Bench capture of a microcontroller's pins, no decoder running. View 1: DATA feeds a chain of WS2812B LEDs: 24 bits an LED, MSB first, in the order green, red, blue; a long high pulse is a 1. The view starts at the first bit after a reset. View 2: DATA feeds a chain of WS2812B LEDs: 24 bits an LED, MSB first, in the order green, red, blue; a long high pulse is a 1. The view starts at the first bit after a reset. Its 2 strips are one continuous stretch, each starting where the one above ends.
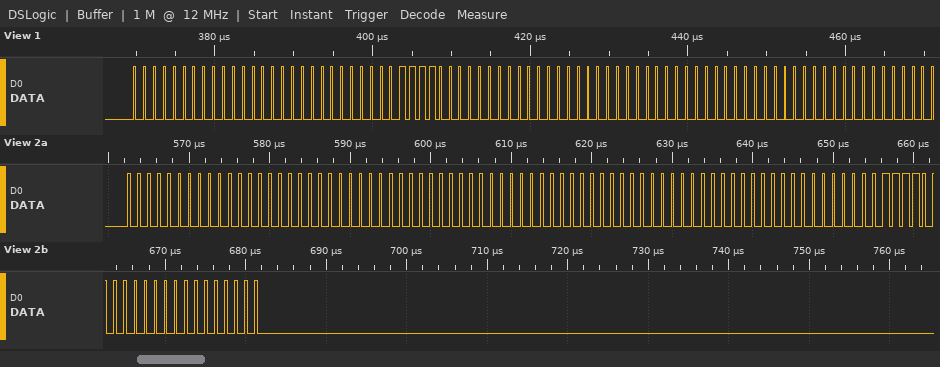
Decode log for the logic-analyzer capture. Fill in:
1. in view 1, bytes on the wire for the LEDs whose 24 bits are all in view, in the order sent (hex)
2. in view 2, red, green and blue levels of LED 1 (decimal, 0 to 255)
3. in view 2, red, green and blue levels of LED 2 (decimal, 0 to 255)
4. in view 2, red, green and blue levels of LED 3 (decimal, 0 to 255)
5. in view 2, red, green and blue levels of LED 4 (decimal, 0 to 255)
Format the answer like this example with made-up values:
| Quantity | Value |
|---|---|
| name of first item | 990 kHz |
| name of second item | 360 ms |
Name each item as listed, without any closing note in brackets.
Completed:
| Quantity | Value |
|---|---|
| in view 1, bytes on the wire for the LEDs whose 24 bits are all in view, in the order sent | 00 00 00 1E 00 00 00 00 00 |
| in view 2, red, green and blue levels of LED 1 | 0, 0, 0 |
| in view 2, red, green and blue levels of LED 2 | 0, 0, 0 |
| in view 2, red, green and blue levels of LED 3 | 0, 0, 0 |
| in view 2, red, green and blue levels of LED 4 | 0, 30, 0 |
